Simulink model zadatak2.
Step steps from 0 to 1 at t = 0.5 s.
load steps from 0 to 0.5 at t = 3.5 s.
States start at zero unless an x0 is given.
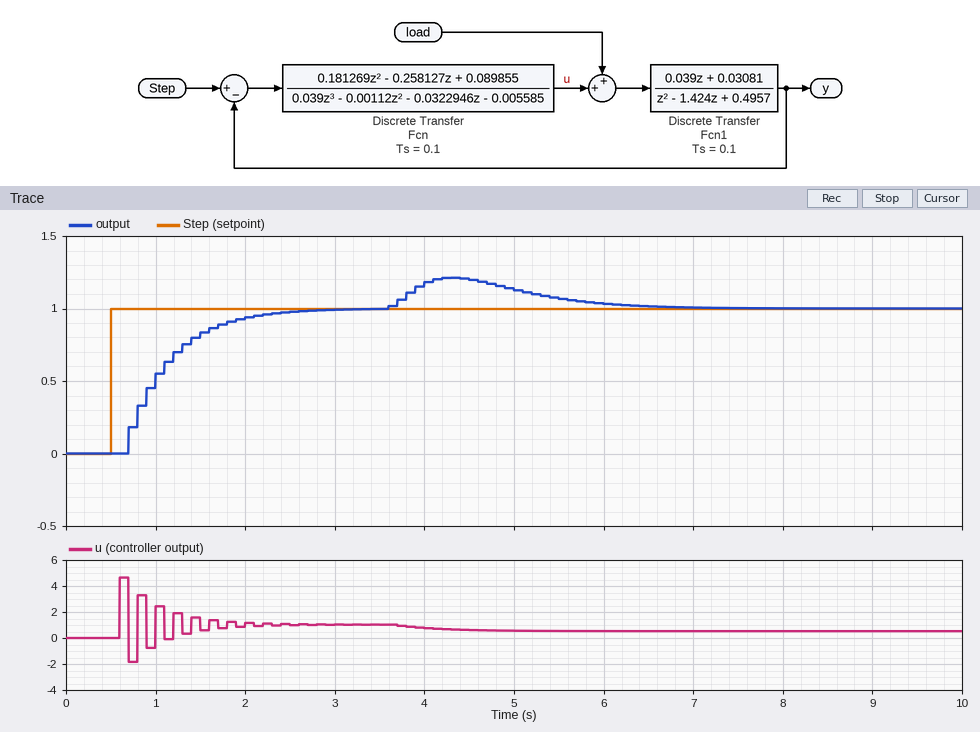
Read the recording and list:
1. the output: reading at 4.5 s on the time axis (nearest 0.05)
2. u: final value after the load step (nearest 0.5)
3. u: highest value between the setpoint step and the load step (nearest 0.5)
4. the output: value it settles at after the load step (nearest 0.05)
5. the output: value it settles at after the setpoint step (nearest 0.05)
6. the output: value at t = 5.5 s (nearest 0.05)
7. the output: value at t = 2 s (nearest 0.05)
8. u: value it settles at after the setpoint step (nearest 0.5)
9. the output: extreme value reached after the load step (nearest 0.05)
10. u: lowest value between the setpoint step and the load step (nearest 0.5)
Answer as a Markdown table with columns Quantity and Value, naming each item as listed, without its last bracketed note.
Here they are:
| Quantity | Value |
|---|---|
| the output: reading at 4.5 s on the time axis | 1.20 |
| u: final value after the load step | 0.5 |
| u: highest value between the setpoint step and the load step | 4.5 |
| the output: value it settles at after the load step | 1.00 |
| the output: value it settles at after the setpoint step | 1.00 |
| the output: value at t = 5.5 s | 1.05 |
| the output: value at t = 2 s | 0.95 |
| u: value it settles at after the setpoint step | 1.0 |
| the output: extreme value reached after the load step | 1.20 |
| u: lowest value between the setpoint step and the load step | -2.0 |
